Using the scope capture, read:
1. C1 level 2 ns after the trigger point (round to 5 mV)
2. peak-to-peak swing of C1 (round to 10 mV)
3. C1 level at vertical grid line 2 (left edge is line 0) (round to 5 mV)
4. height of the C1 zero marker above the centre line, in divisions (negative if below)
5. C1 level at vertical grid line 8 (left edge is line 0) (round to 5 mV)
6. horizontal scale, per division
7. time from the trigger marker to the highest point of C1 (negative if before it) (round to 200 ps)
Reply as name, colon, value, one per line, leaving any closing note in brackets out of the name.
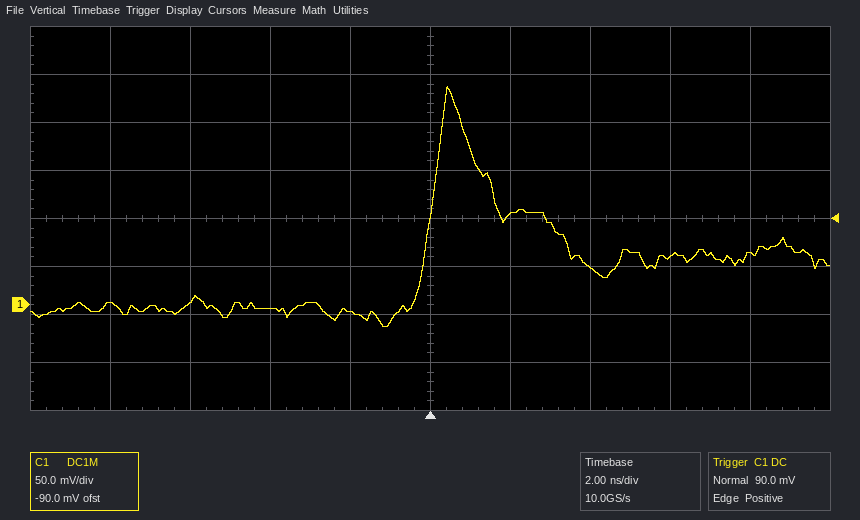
C1 level 2 ns after the trigger point: 95 mV
peak-to-peak swing of C1: 250 mV
C1 level at vertical grid line 2 (left edge is line 0): 5 mV
height of the C1 zero marker above the centre line, in divisions: -1.8 div
C1 level at vertical grid line 8 (left edge is line 0): 50 mV
horizontal scale, per division: 2 ns
time from the trigger marker to the highest point of C1 (negative if before it): +400 ps
